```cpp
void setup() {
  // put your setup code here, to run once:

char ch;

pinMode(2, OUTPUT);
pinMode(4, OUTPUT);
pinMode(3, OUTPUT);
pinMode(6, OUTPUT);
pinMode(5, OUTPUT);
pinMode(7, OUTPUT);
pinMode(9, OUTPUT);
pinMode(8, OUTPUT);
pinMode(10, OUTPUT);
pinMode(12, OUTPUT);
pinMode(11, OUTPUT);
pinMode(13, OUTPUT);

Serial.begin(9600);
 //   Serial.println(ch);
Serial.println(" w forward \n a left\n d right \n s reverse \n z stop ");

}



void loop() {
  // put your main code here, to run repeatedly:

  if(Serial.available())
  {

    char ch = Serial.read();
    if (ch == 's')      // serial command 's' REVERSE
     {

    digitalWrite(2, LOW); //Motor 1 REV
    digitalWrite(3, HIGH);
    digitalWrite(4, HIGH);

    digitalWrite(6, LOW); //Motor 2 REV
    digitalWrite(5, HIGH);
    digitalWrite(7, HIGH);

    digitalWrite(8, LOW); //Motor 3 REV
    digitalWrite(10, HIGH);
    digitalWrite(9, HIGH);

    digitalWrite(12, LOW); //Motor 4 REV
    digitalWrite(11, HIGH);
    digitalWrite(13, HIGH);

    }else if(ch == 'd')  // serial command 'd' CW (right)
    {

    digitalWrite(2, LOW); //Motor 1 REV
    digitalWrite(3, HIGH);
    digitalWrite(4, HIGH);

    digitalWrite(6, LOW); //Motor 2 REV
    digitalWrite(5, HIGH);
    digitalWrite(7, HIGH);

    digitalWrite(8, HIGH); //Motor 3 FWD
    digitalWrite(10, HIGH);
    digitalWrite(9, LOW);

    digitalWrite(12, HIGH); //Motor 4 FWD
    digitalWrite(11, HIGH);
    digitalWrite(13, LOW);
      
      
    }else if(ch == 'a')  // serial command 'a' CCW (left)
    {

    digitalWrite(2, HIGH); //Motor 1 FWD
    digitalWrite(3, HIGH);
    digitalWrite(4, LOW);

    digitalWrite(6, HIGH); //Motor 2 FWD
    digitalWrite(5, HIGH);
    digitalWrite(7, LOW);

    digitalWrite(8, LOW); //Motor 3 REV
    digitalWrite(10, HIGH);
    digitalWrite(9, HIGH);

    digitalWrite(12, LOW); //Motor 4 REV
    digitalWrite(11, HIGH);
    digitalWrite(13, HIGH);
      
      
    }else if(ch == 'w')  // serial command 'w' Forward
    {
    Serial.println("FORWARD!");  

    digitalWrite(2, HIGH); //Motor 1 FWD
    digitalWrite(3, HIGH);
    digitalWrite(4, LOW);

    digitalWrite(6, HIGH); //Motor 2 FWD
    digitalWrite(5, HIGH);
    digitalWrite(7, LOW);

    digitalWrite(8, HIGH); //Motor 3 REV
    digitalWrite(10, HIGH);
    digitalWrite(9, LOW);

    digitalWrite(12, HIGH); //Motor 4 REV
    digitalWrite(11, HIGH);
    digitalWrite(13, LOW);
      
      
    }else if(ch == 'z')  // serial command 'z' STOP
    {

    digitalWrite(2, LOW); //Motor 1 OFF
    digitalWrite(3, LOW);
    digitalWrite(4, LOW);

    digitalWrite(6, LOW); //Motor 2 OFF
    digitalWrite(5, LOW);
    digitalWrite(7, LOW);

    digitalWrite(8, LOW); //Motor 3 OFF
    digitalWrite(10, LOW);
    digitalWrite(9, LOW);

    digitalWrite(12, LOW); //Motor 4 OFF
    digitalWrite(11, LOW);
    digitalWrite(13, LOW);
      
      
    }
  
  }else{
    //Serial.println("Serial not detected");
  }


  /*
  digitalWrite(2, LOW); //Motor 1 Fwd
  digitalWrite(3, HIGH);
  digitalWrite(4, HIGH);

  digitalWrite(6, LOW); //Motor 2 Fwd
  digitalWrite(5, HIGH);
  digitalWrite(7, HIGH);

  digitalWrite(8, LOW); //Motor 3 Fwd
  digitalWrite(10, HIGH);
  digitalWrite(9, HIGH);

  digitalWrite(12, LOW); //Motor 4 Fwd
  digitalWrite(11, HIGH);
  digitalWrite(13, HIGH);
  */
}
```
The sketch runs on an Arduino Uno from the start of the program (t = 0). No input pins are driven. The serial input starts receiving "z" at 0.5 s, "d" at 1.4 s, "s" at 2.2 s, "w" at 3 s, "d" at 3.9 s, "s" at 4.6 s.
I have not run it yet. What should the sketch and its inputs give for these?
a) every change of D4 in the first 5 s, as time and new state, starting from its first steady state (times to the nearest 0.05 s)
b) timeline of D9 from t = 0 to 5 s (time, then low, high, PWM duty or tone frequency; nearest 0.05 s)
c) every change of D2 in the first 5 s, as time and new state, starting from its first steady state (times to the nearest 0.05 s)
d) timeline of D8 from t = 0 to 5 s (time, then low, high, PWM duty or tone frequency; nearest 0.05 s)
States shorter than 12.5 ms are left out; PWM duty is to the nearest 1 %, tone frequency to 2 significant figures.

0 s low; 1.4 s high; 3 s low; 3.9 s high
0 s low; 2.2 s high; 3 s low; 4.6 s high
0 s low; 3 s high; 3.9 s low
0 s low; 1.4 s high; 2.2 s low; 3 s high; 4.6 s low
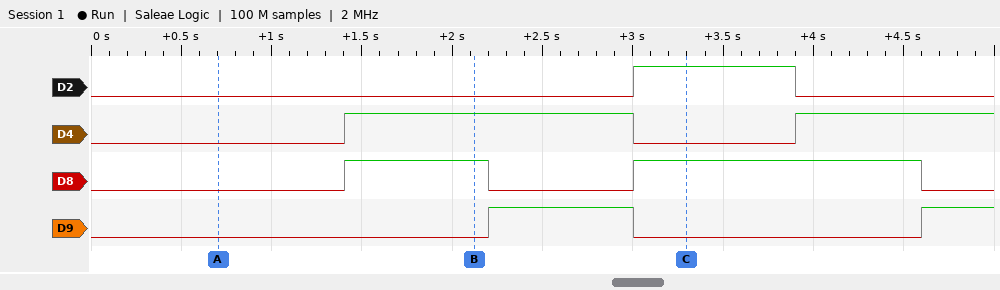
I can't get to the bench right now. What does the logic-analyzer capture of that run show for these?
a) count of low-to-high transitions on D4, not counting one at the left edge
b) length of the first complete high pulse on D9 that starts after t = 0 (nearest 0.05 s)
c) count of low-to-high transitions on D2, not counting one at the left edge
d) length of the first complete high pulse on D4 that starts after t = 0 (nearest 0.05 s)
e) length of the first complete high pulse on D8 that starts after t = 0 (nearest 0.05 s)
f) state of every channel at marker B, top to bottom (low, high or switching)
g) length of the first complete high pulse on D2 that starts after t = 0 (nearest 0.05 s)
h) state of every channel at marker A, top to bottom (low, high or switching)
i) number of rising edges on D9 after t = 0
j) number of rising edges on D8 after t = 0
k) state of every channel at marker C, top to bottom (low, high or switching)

2
0.80 s
1
1.60 s
0.80 s
D2 low, D4 high, D8 high, D9 low
0.90 s
D2 low, D4 low, D8 low, D9 low
2
2
D2 high, D4 low, D8 high, D9 low
